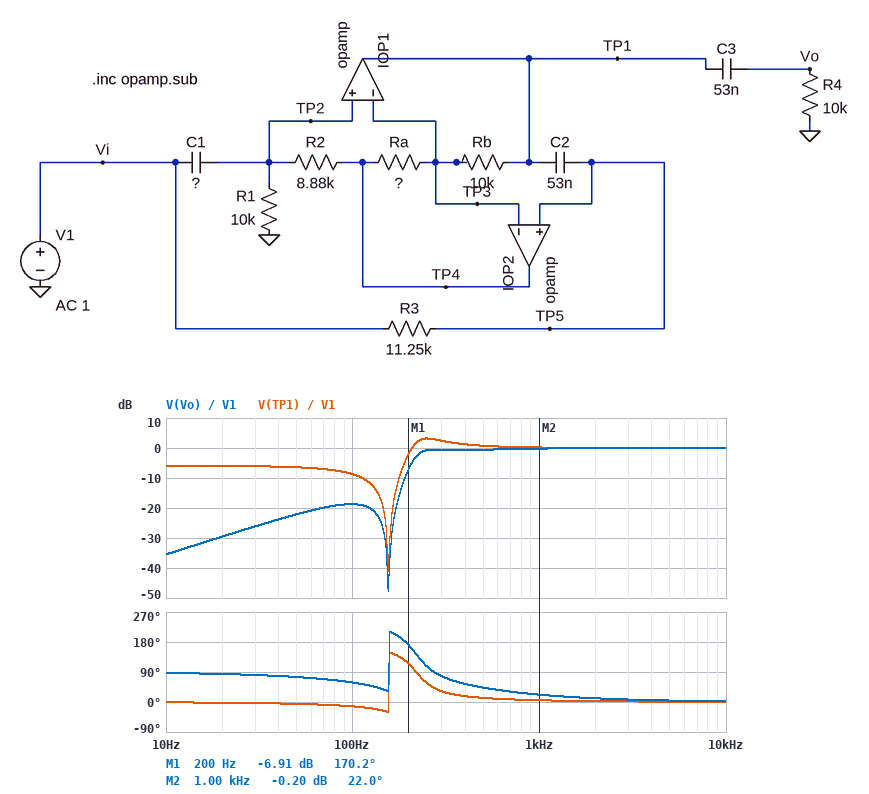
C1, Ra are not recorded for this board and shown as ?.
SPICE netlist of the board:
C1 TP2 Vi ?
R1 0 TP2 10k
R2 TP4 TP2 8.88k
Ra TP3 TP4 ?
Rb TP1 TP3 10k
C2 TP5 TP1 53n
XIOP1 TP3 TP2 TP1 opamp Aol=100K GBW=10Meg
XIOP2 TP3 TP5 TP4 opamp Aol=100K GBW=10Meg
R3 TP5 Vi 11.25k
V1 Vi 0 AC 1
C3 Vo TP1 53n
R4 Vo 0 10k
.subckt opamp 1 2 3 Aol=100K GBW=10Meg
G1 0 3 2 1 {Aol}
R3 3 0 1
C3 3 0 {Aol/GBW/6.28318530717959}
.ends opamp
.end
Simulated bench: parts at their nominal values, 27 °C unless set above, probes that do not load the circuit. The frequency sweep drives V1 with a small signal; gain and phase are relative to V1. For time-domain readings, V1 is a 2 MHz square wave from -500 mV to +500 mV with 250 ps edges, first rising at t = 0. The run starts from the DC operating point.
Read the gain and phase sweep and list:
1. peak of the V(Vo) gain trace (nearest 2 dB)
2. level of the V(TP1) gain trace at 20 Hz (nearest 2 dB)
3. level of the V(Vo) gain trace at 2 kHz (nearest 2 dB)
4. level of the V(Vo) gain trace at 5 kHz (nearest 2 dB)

0 dB
-6 dB
0 dB
0 dB
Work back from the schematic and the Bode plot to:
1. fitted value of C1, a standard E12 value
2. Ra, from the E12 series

180 nF
18 kΩ
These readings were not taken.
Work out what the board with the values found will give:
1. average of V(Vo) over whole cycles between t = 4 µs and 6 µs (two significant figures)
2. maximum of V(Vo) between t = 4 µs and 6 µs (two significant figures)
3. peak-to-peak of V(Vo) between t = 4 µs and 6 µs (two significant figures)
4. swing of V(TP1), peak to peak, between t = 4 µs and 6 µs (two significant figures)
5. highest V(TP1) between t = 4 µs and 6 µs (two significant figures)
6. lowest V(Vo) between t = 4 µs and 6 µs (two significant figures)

490 mV
1.2 V
1.3 V
1.3 V
920 mV
-180 mV
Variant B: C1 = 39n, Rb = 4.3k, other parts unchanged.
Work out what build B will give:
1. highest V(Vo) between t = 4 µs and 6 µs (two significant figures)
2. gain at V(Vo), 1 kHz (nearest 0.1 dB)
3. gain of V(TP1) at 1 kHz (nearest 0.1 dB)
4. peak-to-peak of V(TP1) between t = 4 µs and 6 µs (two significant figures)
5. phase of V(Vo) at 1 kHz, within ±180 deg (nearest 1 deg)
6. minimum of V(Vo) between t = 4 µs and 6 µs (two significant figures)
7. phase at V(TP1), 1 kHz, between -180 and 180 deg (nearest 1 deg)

1.1 V
-0.9 dB
-0.6 dB
1.2 V
57 deg
-120 mV
40 deg
